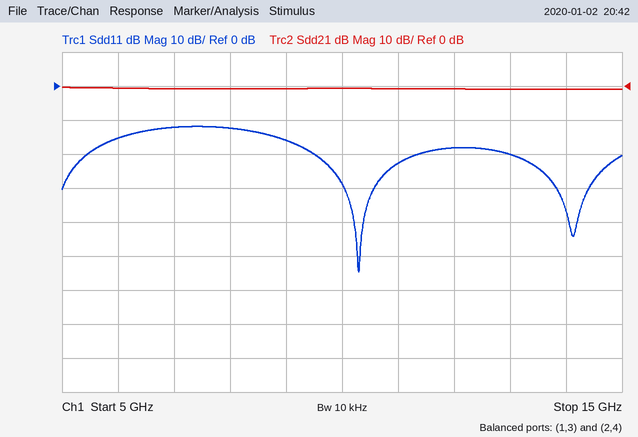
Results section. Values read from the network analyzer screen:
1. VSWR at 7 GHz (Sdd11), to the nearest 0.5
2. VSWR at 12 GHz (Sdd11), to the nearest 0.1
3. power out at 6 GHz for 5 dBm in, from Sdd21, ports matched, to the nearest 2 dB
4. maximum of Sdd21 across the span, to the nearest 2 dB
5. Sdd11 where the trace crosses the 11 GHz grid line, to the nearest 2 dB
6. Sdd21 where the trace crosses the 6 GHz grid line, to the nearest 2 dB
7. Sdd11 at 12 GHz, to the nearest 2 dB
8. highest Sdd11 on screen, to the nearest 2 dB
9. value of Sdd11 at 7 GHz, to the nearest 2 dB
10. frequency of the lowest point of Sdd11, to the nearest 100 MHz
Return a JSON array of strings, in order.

["1.5", "1.3", "4 dBm", "0 dB", "-22 dB", "0 dB", "-18 dB", "-12 dB", "-12 dB", "10.3 GHz"]
